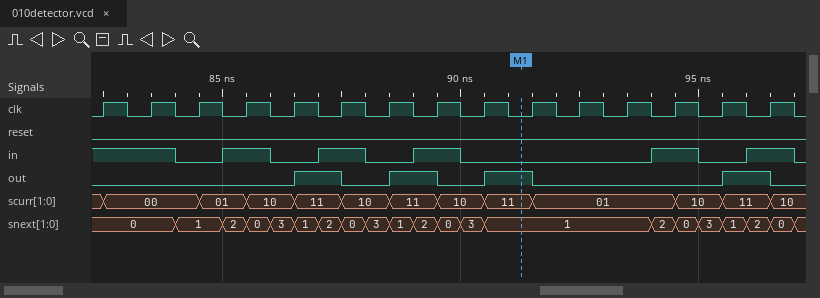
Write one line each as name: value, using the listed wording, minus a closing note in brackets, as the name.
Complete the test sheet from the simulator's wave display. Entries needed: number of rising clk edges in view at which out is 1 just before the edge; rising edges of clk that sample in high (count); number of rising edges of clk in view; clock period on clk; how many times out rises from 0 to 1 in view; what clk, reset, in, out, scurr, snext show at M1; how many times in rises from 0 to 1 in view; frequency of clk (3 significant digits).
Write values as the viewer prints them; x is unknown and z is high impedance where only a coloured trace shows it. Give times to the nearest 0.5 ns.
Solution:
number of rising clk edges in view at which out is 1 just before the edge: 4
rising edges of clk that sample in high: 7
number of rising edges of clk in view: 15
clock period on clk: 1 ns
how many times out rises from 0 to 1 in view: 4
what clk, reset, in, out, scurr, snext show at M1: clk=0, reset=0, in=0, out=1, scurr=11, snext=1
how many times in rises from 0 to 1 in view: 5
frequency of clk: 1.00 GHz
